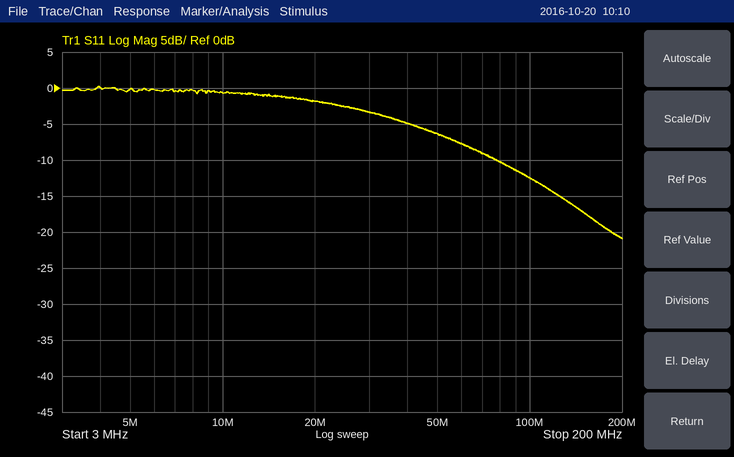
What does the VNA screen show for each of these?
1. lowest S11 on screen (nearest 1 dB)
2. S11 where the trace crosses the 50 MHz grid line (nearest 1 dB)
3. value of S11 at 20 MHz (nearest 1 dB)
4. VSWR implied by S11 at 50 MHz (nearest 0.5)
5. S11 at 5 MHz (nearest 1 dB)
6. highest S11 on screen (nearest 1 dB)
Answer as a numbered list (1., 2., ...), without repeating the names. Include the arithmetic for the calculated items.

1. -21 dB
2. -6 dB
3. -2 dB
4. |Γ| = 10^(-6/20) = 0.5012; VSWR = (1 + 0.5012)/(1 − 0.5012) ≈ 3.0
5. 0 dB
6. 0 dB
